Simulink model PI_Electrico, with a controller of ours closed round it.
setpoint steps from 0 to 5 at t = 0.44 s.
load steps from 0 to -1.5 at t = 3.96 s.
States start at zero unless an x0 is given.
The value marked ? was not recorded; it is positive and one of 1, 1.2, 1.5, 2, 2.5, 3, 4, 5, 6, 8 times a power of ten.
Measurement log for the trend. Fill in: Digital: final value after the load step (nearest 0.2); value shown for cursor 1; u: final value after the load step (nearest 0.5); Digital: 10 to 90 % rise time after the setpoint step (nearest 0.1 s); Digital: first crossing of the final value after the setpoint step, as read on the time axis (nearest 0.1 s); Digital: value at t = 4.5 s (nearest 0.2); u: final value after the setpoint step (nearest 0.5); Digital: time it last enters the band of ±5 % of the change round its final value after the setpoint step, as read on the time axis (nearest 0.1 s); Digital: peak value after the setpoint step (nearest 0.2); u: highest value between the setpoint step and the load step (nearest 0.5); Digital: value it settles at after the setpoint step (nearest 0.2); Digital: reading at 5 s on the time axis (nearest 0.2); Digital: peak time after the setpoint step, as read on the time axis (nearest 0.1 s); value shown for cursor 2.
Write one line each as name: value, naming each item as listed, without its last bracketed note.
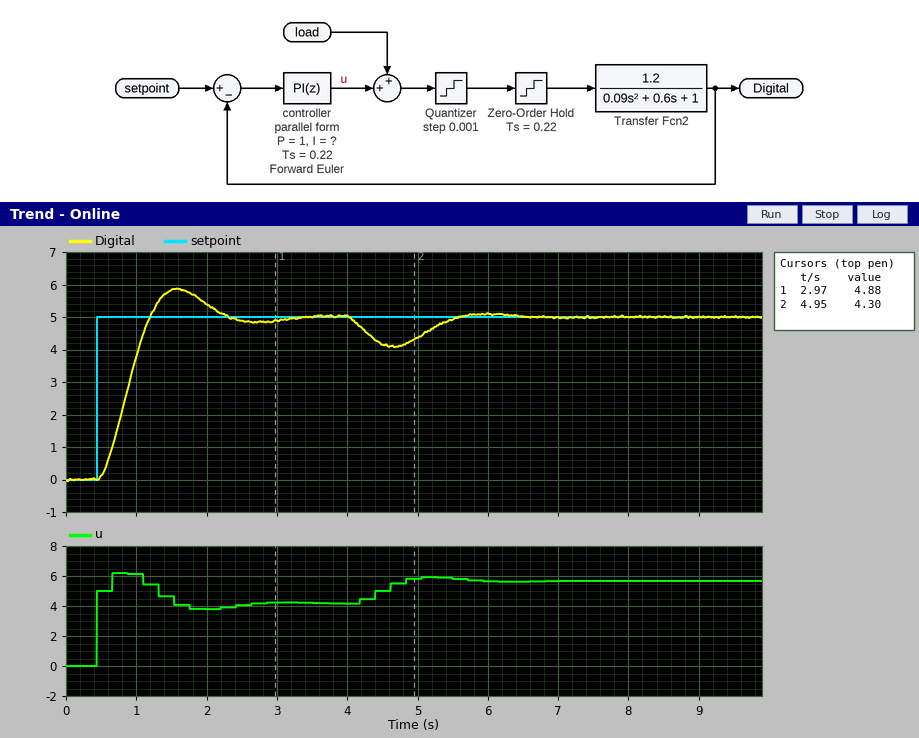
Digital: final value after the load step: 5.0
value shown for cursor 1: 4.88
u: final value after the load step: 5.5
Digital: 10 to 90 % rise time after the setpoint step: 0.5 s
Digital: first crossing of the final value after the setpoint step, as read on the time axis: 1.2 s
Digital: value at t = 4.5 s: 4.2
u: final value after the setpoint step: 4.0
Digital: time it last enters the band of ±5 % of the change round its final value after the setpoint step, as read on the time axis: 2.1 s
Digital: peak value after the setpoint step: 5.8
u: highest value between the setpoint step and the load step: 6.0
Digital: value it settles at after the setpoint step: 5.0
Digital: reading at 5 s on the time axis: 4.4
Digital: peak time after the setpoint step, as read on the time axis: 1.6 s
value shown for cursor 2: 4.30
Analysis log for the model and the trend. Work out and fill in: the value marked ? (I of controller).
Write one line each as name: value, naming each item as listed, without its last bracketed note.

the value marked ?: 2
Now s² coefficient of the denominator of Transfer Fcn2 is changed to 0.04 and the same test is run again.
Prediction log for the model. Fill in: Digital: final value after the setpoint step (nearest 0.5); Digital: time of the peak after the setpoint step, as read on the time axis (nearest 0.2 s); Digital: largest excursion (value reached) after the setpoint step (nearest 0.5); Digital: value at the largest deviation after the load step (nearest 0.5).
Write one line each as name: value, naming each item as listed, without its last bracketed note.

Digital: final value after the setpoint step: 5.0
Digital: time of the peak after the setpoint step, as read on the time axis: 1.8 s
Digital: largest excursion (value reached) after the setpoint step: 5.5
Digital: value at the largest deviation after the load step: 4.0
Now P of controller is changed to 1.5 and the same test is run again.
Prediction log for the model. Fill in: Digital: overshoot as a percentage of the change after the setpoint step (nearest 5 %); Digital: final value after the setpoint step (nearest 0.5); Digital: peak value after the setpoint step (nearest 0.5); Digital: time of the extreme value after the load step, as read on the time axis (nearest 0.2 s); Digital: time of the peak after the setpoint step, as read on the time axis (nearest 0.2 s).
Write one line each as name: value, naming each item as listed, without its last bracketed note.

Digital: overshoot as a percentage of the change after the setpoint step: 15 %
Digital: final value after the setpoint step: 5.0
Digital: peak value after the setpoint step: 5.5
Digital: time of the extreme value after the load step, as read on the time axis: 4.6 s
Digital: time of the peak after the setpoint step, as read on the time axis: 1.2 s
